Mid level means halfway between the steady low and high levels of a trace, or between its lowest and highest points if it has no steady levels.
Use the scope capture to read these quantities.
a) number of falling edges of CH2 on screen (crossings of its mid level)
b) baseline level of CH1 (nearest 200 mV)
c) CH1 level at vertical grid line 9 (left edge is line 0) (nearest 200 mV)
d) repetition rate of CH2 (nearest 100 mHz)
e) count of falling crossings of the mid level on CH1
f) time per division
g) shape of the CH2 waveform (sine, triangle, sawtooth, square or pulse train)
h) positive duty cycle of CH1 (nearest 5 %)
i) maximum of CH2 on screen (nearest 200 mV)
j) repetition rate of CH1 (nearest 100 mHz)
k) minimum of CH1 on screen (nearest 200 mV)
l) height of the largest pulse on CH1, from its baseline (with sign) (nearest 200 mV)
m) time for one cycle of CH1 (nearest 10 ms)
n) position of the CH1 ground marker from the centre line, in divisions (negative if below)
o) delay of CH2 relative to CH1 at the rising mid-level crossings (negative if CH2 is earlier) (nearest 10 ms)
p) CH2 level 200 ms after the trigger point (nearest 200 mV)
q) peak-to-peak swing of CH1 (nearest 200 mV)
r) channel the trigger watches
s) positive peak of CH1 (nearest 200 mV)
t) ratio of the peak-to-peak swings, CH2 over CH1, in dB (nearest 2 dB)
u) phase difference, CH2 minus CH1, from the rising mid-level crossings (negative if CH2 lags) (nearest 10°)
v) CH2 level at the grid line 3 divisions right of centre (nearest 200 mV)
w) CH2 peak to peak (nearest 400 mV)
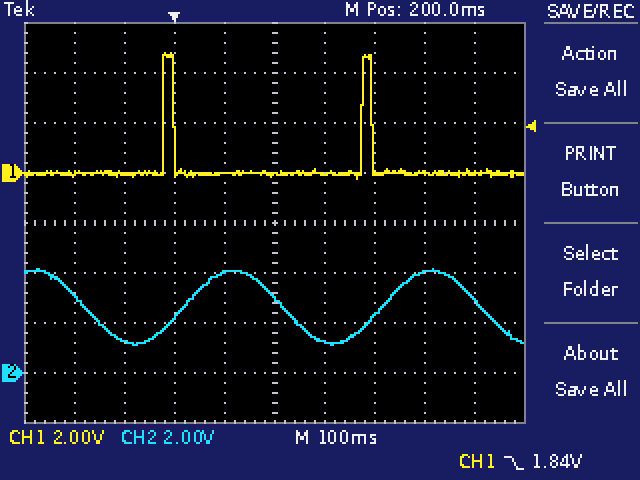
3
0.0 V
0.0 V
2.5 Hz
2
100 ms
sine
5 %
4.2 V
2.5 Hz
-200 mV
+4.8 V
400 ms
+1.0 div
+40 ms
3.0 V
5.0 V
CH1
4.8 V
-4 dB
-40°
4.0 V
3.2 V
